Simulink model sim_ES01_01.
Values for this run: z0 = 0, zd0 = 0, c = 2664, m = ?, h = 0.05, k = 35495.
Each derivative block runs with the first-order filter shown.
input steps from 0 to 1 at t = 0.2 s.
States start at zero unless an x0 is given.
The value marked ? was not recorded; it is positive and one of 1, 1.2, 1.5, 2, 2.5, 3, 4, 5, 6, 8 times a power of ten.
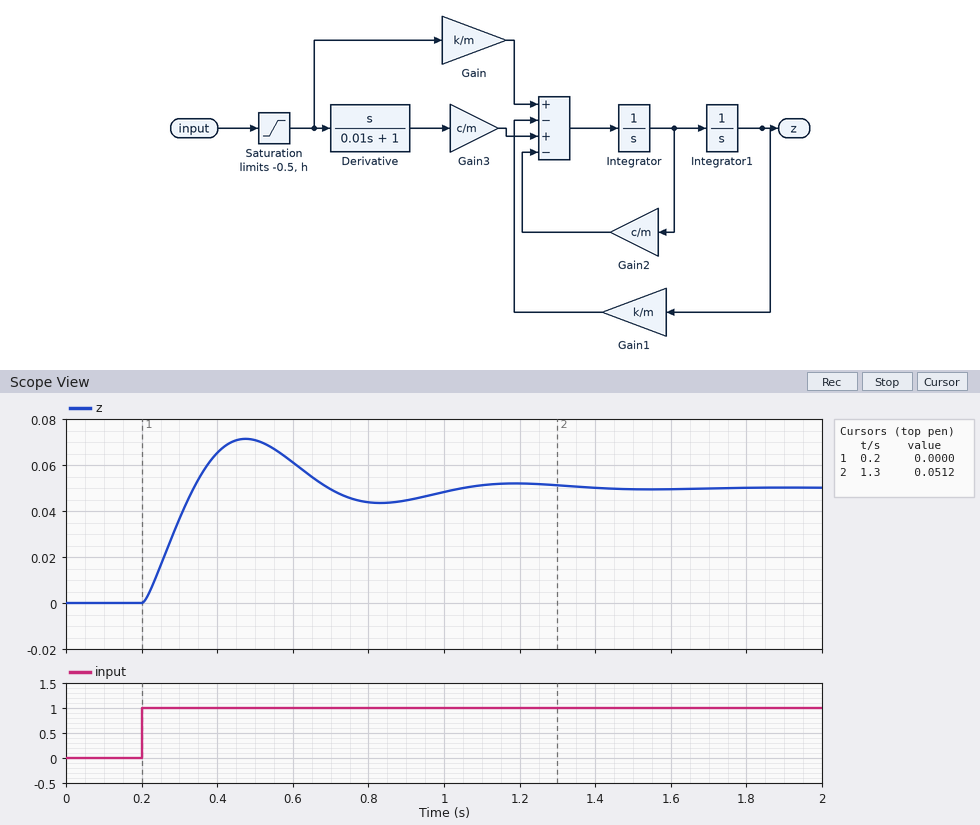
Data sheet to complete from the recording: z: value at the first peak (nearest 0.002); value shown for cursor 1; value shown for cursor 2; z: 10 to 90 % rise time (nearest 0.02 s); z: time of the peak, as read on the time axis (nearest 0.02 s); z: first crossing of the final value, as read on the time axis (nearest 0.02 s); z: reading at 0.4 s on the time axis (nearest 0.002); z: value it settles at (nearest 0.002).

0.072
0.0000
0.0512
0.10 s
0.48 s
0.34 s
0.066
0.050
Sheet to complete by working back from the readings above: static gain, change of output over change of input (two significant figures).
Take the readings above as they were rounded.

0.050
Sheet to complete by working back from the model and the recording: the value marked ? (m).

400
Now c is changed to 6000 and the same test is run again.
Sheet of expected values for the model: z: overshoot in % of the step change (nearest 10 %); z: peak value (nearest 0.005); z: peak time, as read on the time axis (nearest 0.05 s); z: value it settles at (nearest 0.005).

20 %
0.060
0.45 s
0.050
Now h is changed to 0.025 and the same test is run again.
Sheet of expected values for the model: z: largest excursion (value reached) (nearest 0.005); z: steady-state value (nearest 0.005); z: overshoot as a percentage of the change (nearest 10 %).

0.035
0.025
40 %
